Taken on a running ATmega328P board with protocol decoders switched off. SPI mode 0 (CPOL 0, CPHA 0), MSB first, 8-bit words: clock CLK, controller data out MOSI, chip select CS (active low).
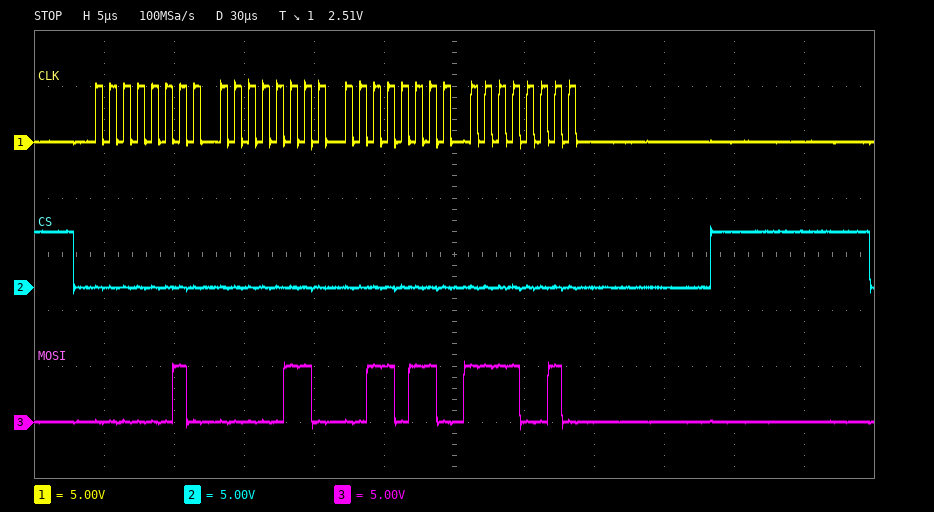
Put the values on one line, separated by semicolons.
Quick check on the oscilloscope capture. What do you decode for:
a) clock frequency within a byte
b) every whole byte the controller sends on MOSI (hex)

1 MHz; 02 06 36 F2
